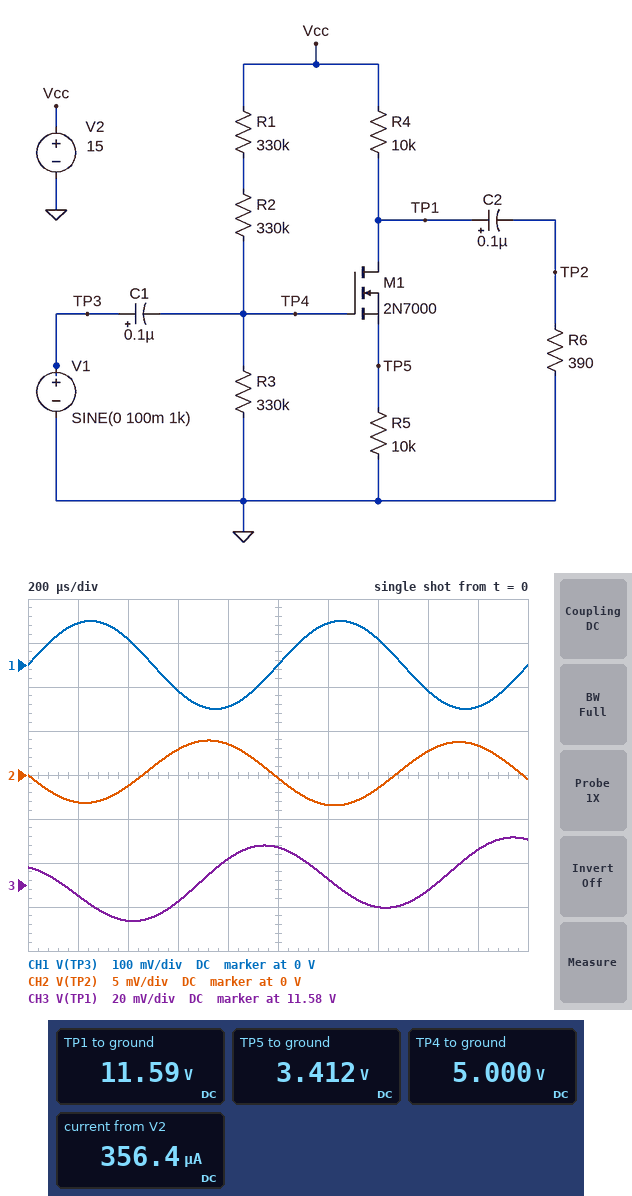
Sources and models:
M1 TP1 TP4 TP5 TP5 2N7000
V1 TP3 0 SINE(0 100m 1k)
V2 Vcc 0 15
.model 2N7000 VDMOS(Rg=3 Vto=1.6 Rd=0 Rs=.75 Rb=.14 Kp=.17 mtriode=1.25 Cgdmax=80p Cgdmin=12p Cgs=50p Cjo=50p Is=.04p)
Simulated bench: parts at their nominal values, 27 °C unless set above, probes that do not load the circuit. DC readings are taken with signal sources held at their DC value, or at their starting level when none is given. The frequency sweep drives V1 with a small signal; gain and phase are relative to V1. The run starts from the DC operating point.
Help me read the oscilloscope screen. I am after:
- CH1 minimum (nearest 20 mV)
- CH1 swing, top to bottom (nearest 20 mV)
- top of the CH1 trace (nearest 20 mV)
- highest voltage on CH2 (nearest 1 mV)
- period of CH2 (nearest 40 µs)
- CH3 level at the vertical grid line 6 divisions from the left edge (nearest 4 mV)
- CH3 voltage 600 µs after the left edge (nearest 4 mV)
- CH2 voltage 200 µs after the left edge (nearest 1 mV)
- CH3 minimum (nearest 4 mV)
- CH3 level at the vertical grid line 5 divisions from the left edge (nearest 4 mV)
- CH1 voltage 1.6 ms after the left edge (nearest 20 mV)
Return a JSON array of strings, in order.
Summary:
["-100 mV", "200 mV", "100 mV", "4 mV", "1.00 ms", "11.584 V", "11.572 V", "-3 mV", "11.564 V", "11.596 V", "-60 mV"]
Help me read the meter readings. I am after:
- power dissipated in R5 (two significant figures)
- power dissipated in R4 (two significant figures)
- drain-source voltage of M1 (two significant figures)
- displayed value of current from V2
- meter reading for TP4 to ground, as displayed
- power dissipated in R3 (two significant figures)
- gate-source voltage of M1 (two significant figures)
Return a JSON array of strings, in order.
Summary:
["1.2 mW", "1.2 mW", "8.2 V", "356.4 µA", "5.000 V", "76 µW", "1.6 V"]
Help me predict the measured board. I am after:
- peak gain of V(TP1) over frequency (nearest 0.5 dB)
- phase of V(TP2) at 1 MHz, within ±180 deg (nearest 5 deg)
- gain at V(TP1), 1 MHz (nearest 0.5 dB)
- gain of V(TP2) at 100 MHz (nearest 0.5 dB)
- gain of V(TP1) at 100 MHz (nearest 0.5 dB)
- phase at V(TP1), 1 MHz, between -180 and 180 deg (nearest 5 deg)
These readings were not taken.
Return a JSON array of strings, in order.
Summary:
["0 dB", "130 deg", "-25.0 dB", "0 dB", "0 dB", "130 deg"]
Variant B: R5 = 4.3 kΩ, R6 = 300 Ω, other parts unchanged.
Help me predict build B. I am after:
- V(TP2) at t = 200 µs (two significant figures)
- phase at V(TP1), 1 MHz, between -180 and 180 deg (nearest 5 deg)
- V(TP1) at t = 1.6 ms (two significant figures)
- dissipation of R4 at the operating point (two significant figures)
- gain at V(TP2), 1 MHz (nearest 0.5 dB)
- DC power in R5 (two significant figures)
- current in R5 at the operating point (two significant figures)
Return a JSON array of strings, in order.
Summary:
["-5.6 mV", "145 deg", "7.2 V", "6.1 mW", "-22.0 dB", "2.6 mW", "780 µA"]
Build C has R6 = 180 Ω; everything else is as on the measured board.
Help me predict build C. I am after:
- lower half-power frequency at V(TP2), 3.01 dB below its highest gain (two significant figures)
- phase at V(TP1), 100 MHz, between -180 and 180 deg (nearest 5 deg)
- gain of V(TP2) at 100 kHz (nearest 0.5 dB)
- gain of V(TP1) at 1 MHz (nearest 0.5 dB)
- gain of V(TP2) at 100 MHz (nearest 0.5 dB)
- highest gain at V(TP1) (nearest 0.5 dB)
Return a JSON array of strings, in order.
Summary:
["29 MHz", "20 deg", "-35.0 dB", "-31.5 dB", "-0.5 dB", "0 dB"]
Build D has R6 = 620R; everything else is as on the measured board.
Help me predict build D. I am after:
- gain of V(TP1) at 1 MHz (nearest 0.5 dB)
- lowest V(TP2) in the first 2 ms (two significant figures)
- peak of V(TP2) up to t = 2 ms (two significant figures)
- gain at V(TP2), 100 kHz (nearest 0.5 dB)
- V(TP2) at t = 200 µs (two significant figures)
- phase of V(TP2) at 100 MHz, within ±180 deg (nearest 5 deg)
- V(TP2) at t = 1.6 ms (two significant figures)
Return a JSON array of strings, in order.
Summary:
["-21.0 dB", "-5.4 mV", "6.1 mV", "-25.0 dB", "-4.9 mV", "5 deg", "4.2 mV"]
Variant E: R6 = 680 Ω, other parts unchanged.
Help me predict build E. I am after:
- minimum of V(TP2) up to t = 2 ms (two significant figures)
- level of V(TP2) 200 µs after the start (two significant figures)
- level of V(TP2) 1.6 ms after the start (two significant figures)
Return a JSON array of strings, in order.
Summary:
["-5.9 mV", "-5.3 mV", "4.6 mV"]
